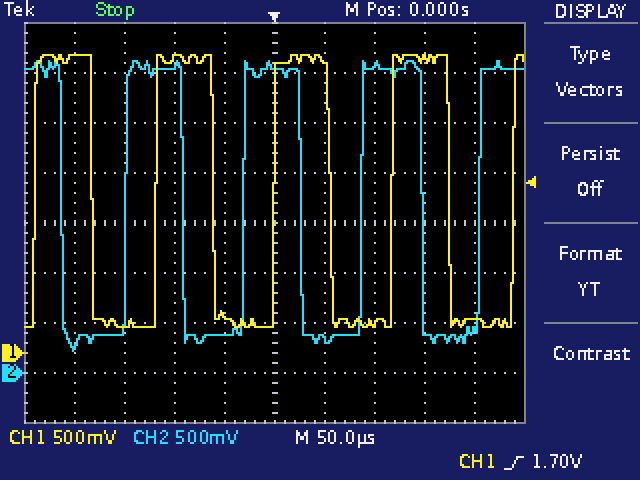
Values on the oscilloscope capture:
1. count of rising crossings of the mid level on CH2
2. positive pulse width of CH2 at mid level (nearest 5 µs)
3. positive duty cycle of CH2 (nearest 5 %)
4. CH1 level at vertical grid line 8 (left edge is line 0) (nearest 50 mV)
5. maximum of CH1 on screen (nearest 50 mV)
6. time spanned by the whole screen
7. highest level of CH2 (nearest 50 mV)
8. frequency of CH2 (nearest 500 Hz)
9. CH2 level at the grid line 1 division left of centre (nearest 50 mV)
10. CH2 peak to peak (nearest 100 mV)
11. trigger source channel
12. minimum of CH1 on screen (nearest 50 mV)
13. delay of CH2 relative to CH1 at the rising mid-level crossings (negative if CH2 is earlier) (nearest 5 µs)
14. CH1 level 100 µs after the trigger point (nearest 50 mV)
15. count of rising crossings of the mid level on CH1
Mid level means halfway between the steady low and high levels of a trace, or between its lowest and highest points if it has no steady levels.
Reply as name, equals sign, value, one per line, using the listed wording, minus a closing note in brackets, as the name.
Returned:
count of rising crossings of the mid level on CH2 = 4
positive pulse width of CH2 at mid level = 60 µs
positive duty cycle of CH2 = 50 %
CH1 level at vertical grid line 8 (left edge is line 0) = 2.95 V
maximum of CH1 on screen = 3.00 V
time spanned by the whole screen = 500 µs
highest level of CH2 = 3.10 V
frequency of CH2 = 8.5 kHz
CH2 level at the grid line 1 division left of centre = 400 mV
CH2 peak to peak = 2.90 V
trigger source channel = CH1
minimum of CH1 on screen = 250 mV
delay of CH2 relative to CH1 at the rising mid-level crossings (negative if CH2 is earlier) = -30 µs
CH1 level 100 µs after the trigger point = 300 mV
count of rising crossings of the mid level on CH1 = 5
